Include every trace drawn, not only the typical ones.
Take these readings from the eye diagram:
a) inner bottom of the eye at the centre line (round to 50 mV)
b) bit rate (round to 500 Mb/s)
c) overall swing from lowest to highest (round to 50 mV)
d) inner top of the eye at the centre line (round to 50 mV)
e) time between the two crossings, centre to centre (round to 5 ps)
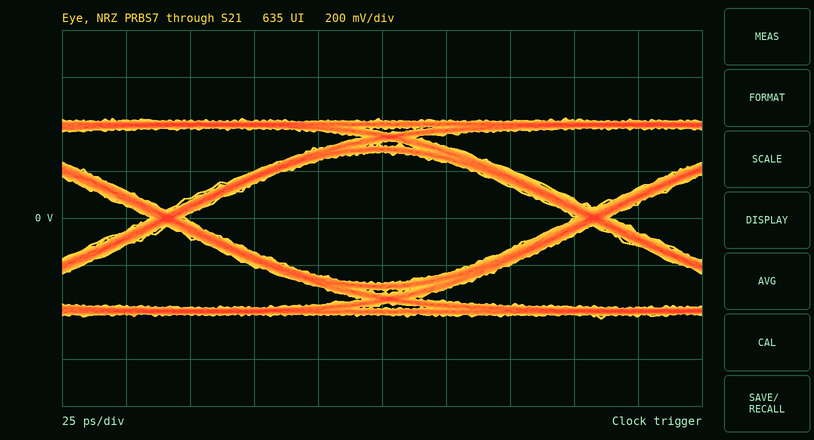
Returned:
-300 mV
6.0 Gb/s
850 mV
300 mV
165 ps
